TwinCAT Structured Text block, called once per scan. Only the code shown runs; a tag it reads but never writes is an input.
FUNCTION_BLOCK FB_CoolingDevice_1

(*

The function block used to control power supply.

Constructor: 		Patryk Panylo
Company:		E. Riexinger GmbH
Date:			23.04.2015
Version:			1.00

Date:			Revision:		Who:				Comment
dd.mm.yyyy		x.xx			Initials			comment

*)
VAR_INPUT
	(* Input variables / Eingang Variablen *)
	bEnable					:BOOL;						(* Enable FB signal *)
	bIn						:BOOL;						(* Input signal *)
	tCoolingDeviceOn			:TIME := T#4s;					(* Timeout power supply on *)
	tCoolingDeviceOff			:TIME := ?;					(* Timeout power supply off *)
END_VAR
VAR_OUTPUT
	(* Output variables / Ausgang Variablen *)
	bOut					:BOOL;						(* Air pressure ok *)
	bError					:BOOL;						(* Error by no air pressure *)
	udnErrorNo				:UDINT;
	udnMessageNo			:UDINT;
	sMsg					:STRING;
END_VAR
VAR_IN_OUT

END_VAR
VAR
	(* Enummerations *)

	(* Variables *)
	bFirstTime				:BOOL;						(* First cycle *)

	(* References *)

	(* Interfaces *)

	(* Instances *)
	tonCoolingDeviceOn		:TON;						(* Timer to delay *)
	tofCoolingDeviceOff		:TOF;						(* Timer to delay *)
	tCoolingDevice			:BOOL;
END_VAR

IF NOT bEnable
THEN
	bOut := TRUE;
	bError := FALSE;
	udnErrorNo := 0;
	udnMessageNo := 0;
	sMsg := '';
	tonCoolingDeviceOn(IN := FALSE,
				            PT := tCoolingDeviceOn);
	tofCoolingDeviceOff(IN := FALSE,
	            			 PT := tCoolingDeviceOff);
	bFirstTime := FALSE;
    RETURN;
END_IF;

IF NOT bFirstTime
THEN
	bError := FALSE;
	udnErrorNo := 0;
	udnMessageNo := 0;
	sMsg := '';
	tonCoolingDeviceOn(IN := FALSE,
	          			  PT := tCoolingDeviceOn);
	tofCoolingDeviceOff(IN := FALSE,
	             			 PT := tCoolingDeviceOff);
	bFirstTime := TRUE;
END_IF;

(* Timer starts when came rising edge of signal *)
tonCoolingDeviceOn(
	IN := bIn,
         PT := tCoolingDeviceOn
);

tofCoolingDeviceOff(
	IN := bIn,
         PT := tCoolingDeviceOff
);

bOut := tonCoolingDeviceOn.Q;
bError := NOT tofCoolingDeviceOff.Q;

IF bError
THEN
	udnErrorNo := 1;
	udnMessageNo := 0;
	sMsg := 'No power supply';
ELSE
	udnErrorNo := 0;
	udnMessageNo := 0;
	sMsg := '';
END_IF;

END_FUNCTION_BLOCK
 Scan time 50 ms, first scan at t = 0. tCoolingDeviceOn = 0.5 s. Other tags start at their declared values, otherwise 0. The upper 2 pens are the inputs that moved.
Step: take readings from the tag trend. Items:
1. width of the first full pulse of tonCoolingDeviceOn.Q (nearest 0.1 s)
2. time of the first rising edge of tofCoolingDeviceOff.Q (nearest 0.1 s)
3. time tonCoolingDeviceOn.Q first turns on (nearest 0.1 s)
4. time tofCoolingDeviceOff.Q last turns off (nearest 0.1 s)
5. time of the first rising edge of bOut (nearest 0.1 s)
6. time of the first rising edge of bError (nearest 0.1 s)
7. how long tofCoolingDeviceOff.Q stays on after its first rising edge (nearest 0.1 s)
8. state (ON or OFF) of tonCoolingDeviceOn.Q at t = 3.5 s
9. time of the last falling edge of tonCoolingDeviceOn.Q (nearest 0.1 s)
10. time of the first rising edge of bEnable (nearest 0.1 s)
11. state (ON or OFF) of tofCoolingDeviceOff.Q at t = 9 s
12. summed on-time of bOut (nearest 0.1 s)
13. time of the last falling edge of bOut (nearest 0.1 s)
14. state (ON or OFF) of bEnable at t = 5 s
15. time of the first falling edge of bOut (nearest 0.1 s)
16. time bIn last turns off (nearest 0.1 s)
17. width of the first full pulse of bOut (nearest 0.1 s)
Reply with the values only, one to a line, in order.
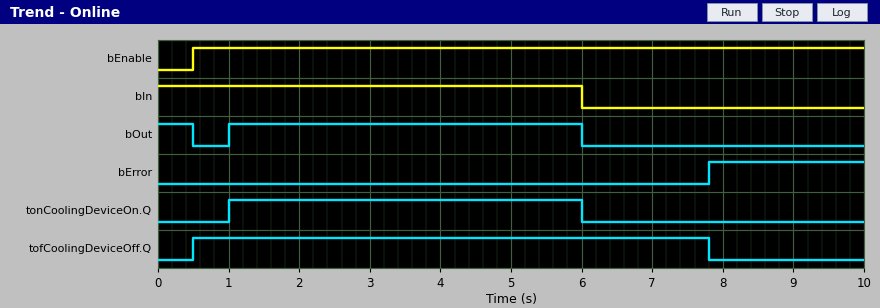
5.0 s
0.5 s
1.0 s
7.8 s
1.0 s
7.8 s
7.3 s
ON
6.0 s
0.5 s
OFF
5.5 s
6.0 s
ON
0.5 s
6.0 s
5.0 s
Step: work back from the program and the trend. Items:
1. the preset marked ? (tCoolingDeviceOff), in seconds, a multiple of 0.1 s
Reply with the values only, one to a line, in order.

1.8 s
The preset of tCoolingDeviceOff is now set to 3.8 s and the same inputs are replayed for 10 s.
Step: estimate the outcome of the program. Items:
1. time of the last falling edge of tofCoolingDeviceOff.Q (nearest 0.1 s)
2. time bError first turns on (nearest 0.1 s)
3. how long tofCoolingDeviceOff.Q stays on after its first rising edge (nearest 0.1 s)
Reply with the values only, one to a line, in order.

9.8 s
9.8 s
9.3 s
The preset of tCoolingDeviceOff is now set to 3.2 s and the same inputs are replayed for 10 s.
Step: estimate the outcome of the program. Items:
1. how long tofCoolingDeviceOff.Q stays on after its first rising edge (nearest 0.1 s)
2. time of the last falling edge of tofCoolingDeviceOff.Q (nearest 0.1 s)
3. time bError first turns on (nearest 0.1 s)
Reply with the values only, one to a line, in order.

8.7 s
9.2 s
9.2 s
